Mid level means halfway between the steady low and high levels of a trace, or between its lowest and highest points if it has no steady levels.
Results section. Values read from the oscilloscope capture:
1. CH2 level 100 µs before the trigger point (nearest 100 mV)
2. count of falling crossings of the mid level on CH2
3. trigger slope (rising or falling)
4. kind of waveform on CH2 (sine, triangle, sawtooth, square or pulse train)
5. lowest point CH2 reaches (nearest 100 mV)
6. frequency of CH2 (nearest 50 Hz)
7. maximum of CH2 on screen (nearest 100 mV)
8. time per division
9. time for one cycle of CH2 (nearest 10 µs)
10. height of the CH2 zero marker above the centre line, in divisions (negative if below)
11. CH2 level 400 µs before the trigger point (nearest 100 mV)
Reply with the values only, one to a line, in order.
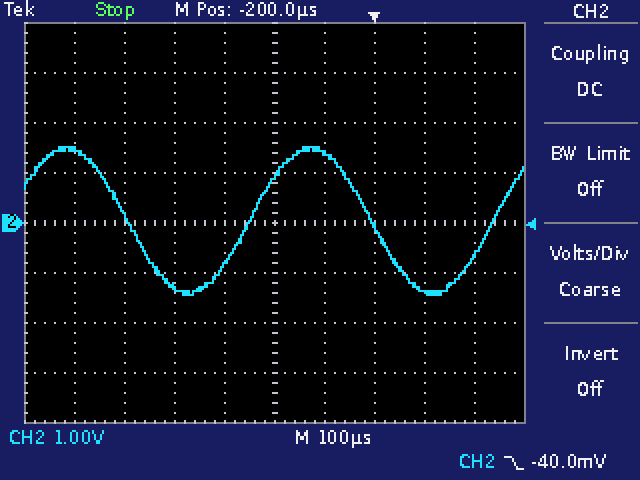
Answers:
1.4 V
2
falling
sine
-1.4 V
2.05 kHz
1.5 V
100 µs
490 µs
0.0 div
-1.3 V
